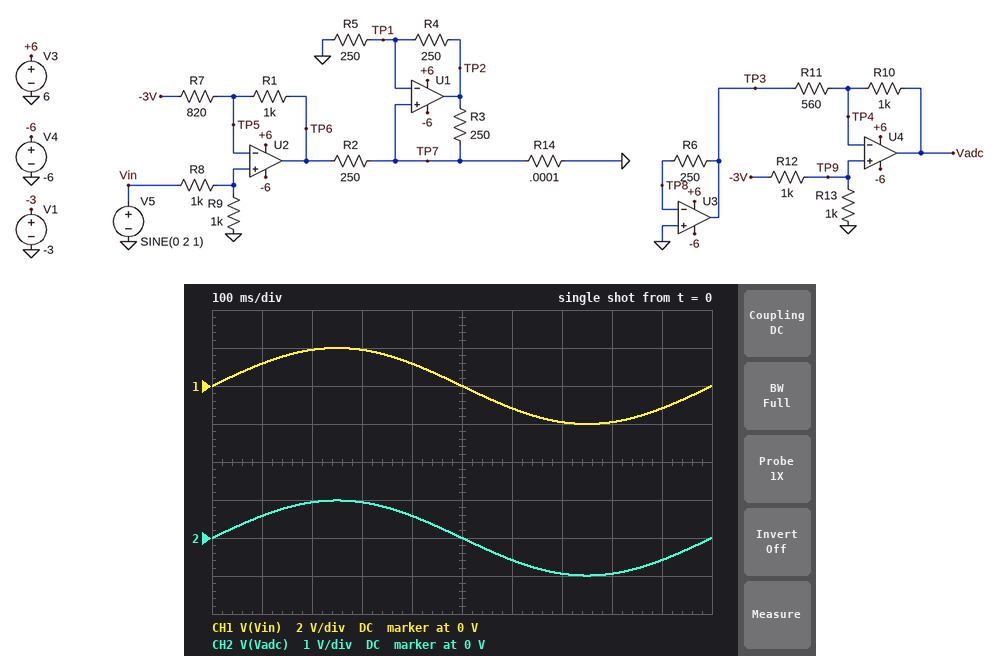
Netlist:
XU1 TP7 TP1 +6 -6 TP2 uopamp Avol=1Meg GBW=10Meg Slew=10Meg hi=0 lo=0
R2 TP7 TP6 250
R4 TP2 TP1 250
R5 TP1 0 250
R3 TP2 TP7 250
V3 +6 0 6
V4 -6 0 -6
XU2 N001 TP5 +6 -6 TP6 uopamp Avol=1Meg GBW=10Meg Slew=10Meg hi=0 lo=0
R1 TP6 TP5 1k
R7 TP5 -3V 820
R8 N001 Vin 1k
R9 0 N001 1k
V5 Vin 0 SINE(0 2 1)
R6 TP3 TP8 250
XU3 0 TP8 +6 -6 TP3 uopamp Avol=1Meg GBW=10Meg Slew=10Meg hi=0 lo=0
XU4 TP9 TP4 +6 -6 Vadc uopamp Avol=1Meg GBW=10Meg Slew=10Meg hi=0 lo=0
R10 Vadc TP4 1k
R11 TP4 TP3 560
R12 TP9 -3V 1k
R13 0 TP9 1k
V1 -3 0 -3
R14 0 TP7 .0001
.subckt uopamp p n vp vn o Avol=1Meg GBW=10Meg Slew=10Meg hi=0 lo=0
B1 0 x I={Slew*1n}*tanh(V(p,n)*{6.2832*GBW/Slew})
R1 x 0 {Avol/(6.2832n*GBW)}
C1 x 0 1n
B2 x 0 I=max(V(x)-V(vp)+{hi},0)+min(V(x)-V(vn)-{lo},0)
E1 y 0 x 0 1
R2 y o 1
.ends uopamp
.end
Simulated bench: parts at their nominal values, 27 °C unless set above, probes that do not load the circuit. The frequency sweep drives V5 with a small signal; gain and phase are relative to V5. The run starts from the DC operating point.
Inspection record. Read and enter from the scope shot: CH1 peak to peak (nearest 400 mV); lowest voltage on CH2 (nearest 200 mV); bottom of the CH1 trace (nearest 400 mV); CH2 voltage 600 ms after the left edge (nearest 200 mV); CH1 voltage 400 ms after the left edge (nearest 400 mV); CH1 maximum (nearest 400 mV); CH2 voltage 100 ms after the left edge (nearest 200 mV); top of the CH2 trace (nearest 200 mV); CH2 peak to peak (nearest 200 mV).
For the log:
4.0 V
-1.0 V
-2.0 V
-600 mV
1.2 V
2.0 V
600 mV
1.0 V
2.0 V
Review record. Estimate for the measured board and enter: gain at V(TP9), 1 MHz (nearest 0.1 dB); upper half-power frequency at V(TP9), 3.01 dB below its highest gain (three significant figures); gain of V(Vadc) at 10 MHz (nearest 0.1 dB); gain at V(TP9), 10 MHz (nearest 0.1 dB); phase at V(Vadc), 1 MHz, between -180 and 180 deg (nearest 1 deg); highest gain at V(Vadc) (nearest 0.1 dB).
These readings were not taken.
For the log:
-15.1 dB
7.35 MHz
-20.1 dB
-19.6 dB
-23 deg
-6.1 dB
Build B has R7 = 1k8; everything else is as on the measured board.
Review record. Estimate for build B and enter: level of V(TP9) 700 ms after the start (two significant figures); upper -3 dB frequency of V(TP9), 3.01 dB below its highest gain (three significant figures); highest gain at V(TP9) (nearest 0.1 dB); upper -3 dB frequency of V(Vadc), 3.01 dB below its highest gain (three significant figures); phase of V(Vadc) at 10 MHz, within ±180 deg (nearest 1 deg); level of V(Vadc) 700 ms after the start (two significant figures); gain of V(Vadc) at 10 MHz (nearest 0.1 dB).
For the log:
-250 mV
7.88 MHz
-17.6 dB
3.08 MHz
-122 deg
-700 mV
-22.3 dB
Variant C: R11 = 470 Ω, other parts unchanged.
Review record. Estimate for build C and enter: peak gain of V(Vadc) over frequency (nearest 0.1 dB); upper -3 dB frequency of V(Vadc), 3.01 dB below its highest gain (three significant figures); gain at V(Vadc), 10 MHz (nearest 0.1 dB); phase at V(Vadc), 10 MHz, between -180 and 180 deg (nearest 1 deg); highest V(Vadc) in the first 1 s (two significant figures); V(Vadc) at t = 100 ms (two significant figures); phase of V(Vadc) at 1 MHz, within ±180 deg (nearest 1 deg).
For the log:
-5.1 dB
2.77 MHz
-20.0 dB
-126 deg
1.1 V
650 mV
-25 deg
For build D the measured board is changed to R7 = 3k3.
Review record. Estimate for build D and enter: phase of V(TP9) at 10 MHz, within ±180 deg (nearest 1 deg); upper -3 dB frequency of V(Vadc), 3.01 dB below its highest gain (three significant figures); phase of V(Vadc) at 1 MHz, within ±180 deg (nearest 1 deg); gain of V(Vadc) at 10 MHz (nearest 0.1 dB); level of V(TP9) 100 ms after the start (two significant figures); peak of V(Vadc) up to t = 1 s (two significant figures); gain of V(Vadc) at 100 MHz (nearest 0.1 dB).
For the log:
-50 deg
3.12 MHz
-22 deg
-24.9 dB
110 mV
530 mV
-62.1 dB
